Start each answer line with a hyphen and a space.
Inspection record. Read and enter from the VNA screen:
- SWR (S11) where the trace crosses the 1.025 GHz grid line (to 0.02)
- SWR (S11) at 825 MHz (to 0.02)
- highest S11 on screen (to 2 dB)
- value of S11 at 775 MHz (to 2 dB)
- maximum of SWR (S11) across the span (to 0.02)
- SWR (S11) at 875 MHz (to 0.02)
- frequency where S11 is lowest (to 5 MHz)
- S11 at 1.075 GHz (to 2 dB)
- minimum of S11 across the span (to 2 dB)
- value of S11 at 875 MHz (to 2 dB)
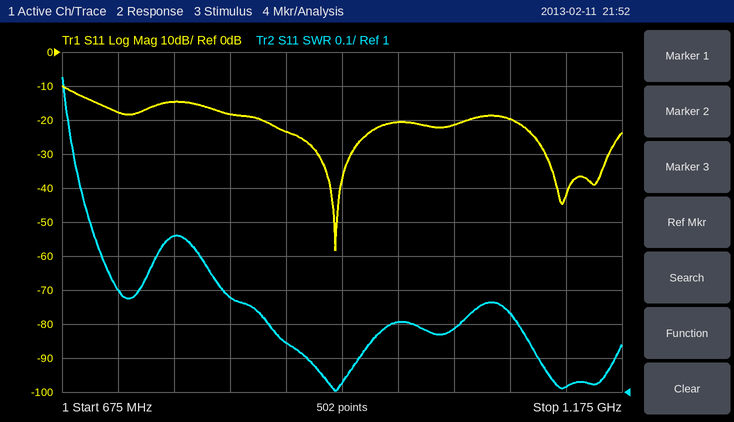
- 1.18
- 1.28
- -10 dB
- -14 dB
- 1.92
- 1.14
- 920 MHz
- -20 dB
- -58 dB
- -24 dB
